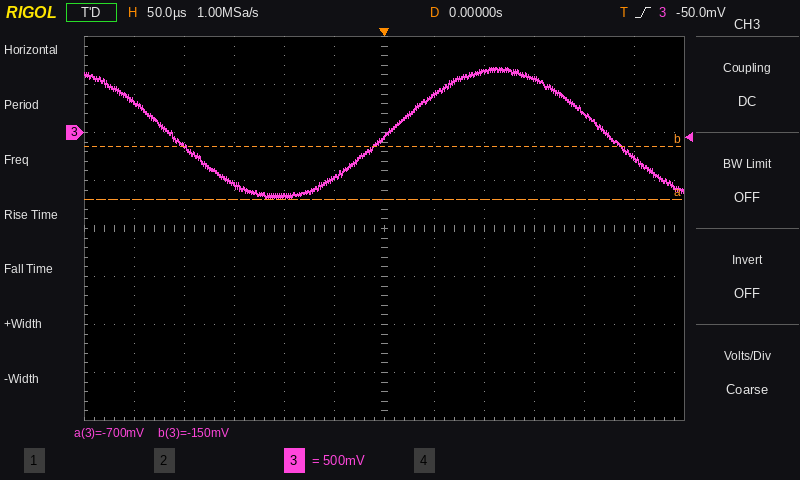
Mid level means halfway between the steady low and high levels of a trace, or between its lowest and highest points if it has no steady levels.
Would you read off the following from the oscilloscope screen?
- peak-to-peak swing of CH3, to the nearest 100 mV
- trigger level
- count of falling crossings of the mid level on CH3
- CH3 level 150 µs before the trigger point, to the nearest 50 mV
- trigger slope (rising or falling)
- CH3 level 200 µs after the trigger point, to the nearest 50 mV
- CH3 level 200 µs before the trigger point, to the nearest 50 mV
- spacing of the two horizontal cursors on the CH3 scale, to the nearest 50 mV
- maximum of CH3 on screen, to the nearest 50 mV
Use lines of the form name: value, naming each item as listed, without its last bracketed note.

peak-to-peak swing of CH3, to the nearest 100 mV: 1.40 V
trigger level: -50.0 mV
count of falling crossings of the mid level on CH3: 2
CH3 level 150 µs before the trigger point, to the nearest 50 mV: -550 mV
trigger slope: rising
CH3 level 200 µs after the trigger point, to the nearest 50 mV: 200 mV
CH3 level 200 µs before the trigger point, to the nearest 50 mV: -150 mV
spacing of the two horizontal cursors on the CH3 scale, to the nearest 50 mV: 550 mV
maximum of CH3 on screen, to the nearest 50 mV: 700 mV
